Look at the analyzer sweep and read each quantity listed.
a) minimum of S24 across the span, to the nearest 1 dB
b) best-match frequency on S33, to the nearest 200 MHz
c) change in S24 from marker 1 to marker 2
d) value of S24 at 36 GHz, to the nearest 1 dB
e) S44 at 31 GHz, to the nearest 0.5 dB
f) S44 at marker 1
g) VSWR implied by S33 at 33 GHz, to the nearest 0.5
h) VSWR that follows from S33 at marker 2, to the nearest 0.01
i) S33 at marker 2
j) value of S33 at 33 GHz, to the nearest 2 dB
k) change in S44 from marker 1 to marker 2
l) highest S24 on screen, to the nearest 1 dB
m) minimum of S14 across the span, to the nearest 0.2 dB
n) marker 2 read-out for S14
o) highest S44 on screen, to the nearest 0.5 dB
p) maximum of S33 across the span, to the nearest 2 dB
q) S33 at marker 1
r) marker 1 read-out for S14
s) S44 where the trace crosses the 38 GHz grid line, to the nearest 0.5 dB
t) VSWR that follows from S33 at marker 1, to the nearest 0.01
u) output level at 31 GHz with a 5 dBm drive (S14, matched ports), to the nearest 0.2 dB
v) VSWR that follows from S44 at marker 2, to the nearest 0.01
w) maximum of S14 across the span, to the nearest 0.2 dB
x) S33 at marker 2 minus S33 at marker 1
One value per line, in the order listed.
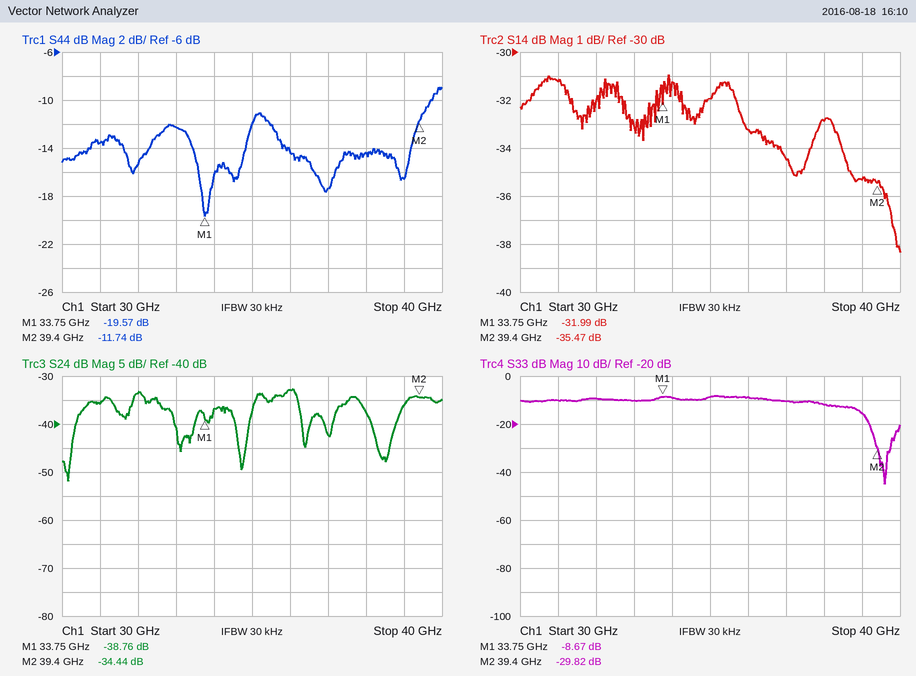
-52 dB
39.6 GHz
4.32 dB
-33 dB
-13.5 dB
-19.57 dB
2.0
1.07
-29.82 dB
-10 dB
7.83 dB
-33 dB
-38.4 dB
-35.47 dB
-9.0 dB
-8 dB
-8.67 dB
-31.99 dB
-14.5 dB
2.17
-26.2 dBm
1.70
-31.0 dB
-21.15 dB
